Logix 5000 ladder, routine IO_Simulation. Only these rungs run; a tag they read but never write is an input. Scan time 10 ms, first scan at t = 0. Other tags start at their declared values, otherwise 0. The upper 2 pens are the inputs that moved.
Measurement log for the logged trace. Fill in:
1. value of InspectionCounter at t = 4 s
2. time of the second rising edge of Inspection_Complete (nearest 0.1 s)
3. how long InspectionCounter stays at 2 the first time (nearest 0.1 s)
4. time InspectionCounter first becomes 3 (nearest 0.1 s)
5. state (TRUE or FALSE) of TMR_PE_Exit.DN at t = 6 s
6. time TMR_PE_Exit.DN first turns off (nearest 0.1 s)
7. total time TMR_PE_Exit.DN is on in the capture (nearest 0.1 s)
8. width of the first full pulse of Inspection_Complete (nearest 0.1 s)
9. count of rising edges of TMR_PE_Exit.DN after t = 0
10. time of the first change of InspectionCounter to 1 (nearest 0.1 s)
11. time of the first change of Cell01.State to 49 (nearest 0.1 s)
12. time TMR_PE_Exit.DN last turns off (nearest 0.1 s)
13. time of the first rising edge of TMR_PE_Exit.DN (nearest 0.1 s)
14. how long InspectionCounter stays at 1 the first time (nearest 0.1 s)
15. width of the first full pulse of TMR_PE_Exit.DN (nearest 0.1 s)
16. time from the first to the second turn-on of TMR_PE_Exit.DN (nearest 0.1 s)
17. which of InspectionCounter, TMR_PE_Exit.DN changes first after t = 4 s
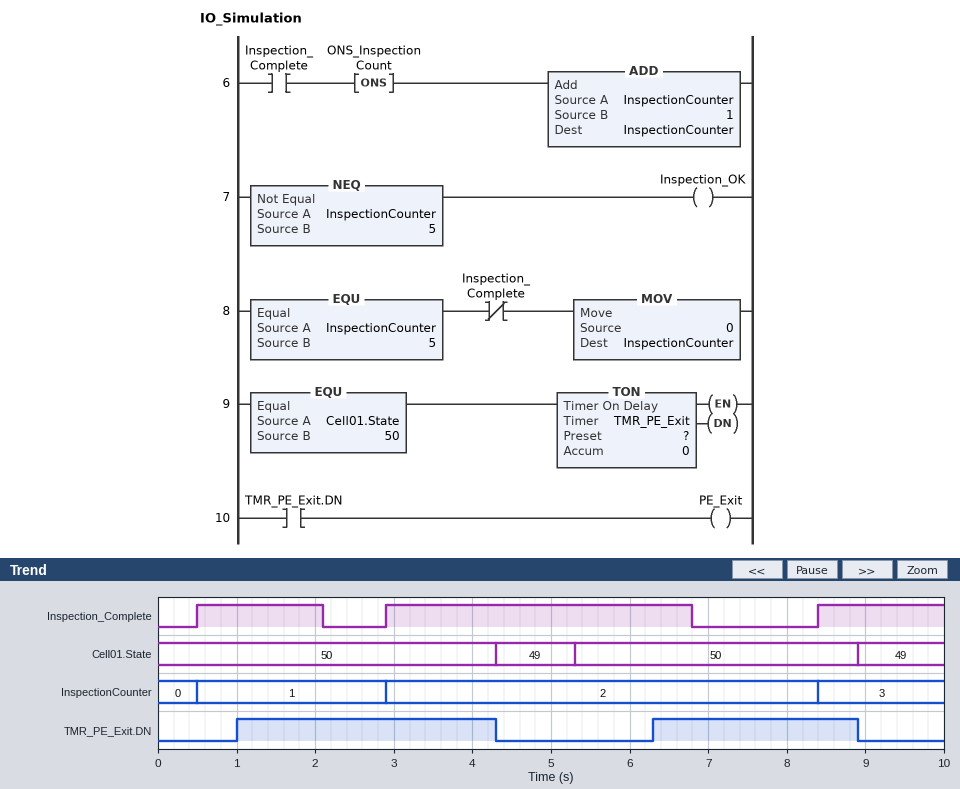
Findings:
2
2.9 s
5.5 s
8.4 s
FALSE
4.3 s
5.9 s
1.6 s
2
0.5 s
4.3 s
8.9 s
1.0 s
2.4 s
3.3 s
5.3 s
TMR_PE_Exit.DN
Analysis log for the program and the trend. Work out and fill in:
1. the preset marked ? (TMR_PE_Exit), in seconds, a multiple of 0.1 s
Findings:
1.0 s
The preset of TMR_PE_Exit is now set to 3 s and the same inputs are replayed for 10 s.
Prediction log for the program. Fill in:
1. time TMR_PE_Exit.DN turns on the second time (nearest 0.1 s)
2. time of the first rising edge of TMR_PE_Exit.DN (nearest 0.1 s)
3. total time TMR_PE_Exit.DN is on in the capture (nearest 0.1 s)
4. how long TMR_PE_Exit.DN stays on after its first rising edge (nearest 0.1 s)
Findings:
8.3 s
3.0 s
1.9 s
1.3 s
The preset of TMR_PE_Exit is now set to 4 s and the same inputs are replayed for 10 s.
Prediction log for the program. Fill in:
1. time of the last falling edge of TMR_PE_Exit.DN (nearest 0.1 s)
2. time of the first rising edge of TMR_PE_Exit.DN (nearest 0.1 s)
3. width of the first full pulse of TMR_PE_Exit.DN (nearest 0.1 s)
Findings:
4.3 s
4.0 s
0.3 s
